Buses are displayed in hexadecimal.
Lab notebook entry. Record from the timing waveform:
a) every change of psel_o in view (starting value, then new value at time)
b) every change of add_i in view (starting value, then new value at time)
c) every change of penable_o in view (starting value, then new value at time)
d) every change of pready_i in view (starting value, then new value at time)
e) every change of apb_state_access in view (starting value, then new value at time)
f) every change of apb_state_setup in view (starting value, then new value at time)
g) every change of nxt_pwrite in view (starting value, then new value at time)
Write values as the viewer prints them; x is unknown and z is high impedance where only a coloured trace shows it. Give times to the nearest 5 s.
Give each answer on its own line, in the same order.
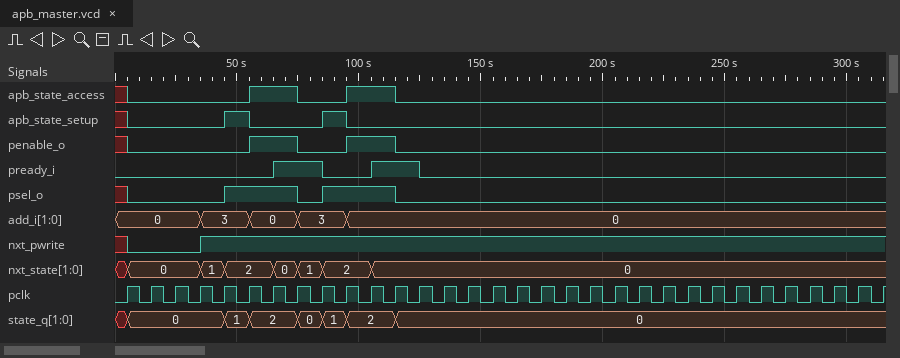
x, 0 at 5 s, 1 at 45 s, 0 at 75 s, 1 at 85 s, 0 at 115 s
0, 3 at 35 s, 0 at 55 s, 3 at 75 s, 0 at 95 s
x, 0 at 5 s, 1 at 55 s, 0 at 75 s, 1 at 95 s, 0 at 115 s
0, 1 at 65 s, 0 at 85 s, 1 at 105 s, 0 at 125 s
x, 0 at 5 s, 1 at 55 s, 0 at 75 s, 1 at 95 s, 0 at 115 s
x, 0 at 5 s, 1 at 45 s, 0 at 55 s, 1 at 85 s, 0 at 95 s
x, 0 at 5 s, 1 at 35 s
